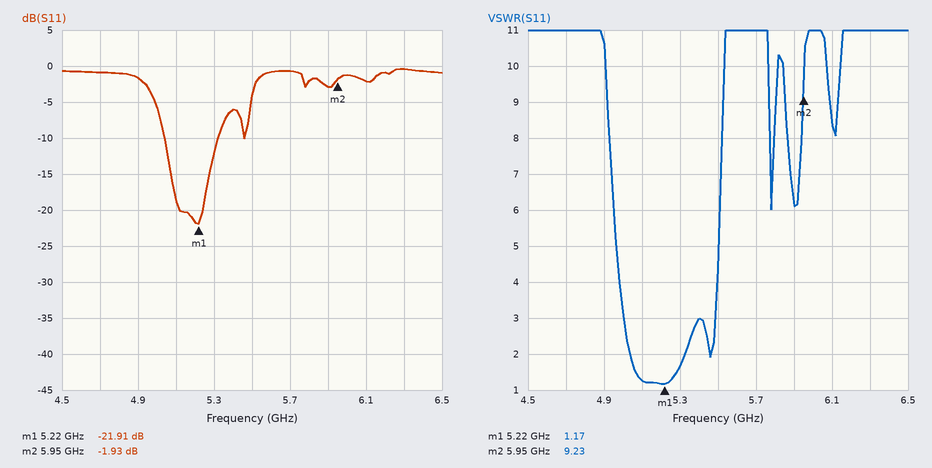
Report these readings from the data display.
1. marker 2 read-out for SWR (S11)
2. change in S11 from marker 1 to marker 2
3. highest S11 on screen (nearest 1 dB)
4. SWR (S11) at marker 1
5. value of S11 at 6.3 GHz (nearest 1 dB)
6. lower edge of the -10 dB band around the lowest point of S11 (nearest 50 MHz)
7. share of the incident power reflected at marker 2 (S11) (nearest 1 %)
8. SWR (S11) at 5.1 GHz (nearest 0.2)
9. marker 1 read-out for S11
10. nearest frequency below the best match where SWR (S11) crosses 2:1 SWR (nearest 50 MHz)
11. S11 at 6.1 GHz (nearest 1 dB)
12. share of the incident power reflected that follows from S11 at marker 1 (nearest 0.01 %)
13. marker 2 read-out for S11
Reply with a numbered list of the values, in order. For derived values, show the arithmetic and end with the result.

1. 9.23
2. -1.93 − (-21.91) = 19.98 dB
3. 0 dB
4. 1.17
5. 0 dB
6. 5.05 GHz
7. 10^(-1.93/10) ≈ 64 %
8. 1.2
9. -21.91 dB
10. 5.05 GHz
11. -2 dB
12. 10^(-21.91/10) ≈ 0.64 %
13. -1.93 dB
